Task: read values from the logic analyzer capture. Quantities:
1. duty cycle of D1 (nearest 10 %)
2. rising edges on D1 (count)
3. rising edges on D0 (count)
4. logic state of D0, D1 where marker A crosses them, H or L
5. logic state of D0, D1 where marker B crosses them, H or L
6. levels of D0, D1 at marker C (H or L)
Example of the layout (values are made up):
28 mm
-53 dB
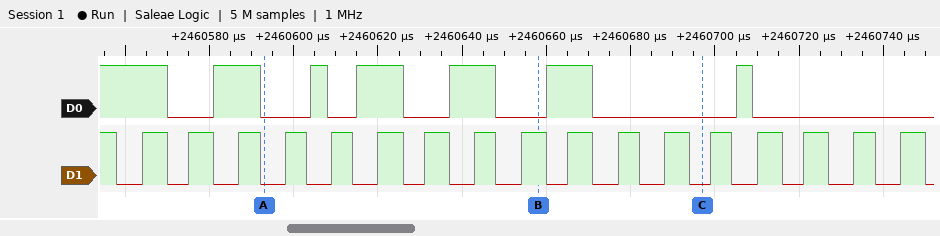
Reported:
50 %
17
6
D0=L, D1=L
D0=L, D1=H
D0=L, D1=L
